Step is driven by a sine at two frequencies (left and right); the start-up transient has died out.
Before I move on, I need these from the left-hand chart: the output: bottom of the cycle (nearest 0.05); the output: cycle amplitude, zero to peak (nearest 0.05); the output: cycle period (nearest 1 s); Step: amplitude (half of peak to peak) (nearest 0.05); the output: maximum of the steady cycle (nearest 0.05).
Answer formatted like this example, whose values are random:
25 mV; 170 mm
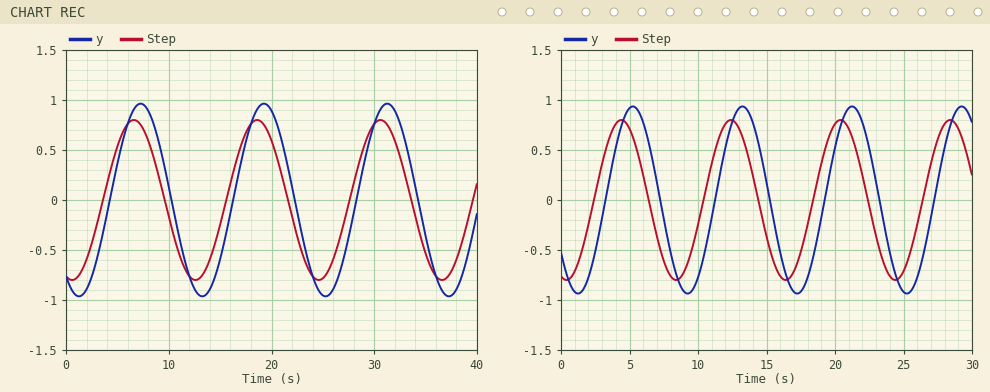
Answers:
-0.95; 0.95; 12 s; 0.80; 0.95
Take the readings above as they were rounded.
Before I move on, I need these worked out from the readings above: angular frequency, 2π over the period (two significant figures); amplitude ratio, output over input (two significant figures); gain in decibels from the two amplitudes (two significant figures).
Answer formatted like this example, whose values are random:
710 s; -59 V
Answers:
0.52 rad/s; 1.2; 1.5 dB
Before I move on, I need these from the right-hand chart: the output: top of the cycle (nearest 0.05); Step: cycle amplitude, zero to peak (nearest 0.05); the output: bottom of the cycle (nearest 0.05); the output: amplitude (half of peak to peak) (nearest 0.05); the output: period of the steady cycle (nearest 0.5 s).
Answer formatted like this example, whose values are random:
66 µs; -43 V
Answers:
0.95; 0.80; -0.95; 0.95; 8.0 s
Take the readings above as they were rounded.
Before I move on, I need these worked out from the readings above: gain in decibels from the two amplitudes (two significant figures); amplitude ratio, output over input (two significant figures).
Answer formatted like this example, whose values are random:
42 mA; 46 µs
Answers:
1.5 dB; 1.2
